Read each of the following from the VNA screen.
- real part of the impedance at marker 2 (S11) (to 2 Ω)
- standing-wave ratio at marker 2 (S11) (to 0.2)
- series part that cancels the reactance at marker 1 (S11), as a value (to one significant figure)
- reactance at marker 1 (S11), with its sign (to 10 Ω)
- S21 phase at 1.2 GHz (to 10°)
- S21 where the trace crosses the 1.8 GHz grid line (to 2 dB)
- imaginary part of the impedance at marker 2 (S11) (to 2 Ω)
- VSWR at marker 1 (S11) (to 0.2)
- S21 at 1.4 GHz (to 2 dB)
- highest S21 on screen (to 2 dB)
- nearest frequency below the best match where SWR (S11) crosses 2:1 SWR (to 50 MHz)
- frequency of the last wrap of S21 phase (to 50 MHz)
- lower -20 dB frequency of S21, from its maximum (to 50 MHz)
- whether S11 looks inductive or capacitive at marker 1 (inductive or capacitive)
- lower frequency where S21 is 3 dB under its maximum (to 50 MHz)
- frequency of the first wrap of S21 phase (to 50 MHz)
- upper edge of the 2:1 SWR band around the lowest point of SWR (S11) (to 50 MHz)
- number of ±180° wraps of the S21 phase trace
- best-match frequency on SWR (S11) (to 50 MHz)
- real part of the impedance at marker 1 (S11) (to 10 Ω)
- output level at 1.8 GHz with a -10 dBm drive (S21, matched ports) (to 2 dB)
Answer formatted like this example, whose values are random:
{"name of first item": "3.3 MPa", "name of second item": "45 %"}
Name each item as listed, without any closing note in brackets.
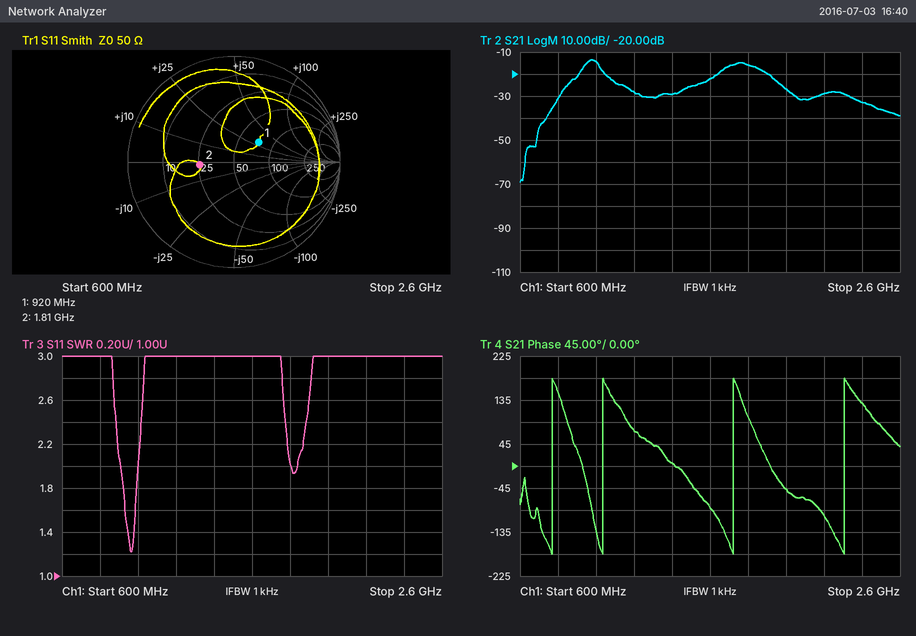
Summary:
{"real part of the impedance at marker 2 (S11)": "26 Ω", "standing-wave ratio at marker 2 (S11)": "2.0", "series part that cancels the reactance at marker 1 (S11), as a value": "6 pF", "reactance at marker 1 (S11), with its sign": "+30 Ω", "S21 phase at 1.2 GHz": "70°", "S21 where the trace crosses the 1.8 GHz grid line": "-16 dB", "imaginary part of the impedance at marker 2 (S11)": "-2 Ω", "VSWR at marker 1 (S11)": "1.8", "S21 at 1.4 GHz": "-30 dB", "highest S21 on screen": "-14 dB", "nearest frequency below the best match where SWR (S11) crosses 2:1 SWR": "900 MHz", "frequency of the last wrap of S21 phase": "2.30 GHz", "lower -20 dB frequency of S21, from its maximum": "800 MHz", "whether S11 looks inductive or capacitive at marker 1": "inductive", "lower frequency where S21 is 3 dB under its maximum": "950 MHz", "frequency of the first wrap of S21 phase": "750 MHz", "upper edge of the 2:1 SWR band around the lowest point of SWR (S11)": "1.00 GHz", "number of ±180° wraps of the S21 phase trace": "4", "best-match frequency on SWR (S11)": "950 MHz", "real part of the impedance at marker 1 (S11)": "70 Ω", "output level at 1.8 GHz with a -10 dBm drive (S21, matched ports)": "-26 dBm"}
